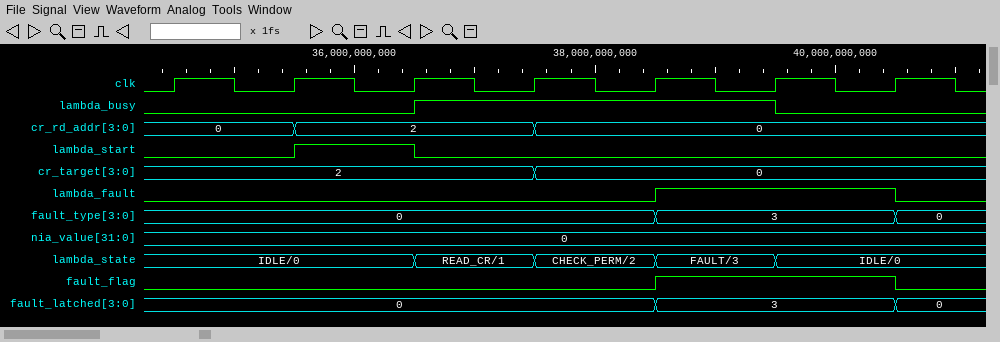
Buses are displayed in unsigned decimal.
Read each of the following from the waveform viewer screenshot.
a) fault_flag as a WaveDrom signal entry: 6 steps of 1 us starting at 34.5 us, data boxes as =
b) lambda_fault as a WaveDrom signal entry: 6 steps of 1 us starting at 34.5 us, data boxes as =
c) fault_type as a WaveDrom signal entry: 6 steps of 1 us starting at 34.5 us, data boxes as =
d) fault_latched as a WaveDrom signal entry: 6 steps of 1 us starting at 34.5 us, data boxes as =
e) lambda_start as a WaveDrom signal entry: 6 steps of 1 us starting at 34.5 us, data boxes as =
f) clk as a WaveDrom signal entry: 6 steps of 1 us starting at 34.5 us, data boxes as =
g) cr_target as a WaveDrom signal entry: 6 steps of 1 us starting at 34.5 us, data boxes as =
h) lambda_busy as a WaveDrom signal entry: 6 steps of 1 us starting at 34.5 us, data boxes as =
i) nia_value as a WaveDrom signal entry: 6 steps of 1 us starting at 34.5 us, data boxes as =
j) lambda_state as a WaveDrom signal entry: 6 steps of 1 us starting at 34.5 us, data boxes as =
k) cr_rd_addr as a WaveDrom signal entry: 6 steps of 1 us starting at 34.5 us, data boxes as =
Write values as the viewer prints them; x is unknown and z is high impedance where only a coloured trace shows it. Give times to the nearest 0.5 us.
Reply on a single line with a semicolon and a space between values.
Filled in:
{name: 'fault_flag', wave: '0...1.'}; {name: 'lambda_fault', wave: '0...1.'}; {name: 'fault_type', wave: '=...=.', data: '0 3'}; {name: 'fault_latched', wave: '=...=.', data: '0 3'}; {name: 'lambda_start', wave: '010...'}; {name: 'clk', wave: 'p.....'}; {name: 'cr_target', wave: '=..=..', data: '2 0'}; {name: 'lambda_busy', wave: '0.1..0'}; {name: 'nia_value', wave: '=.....', data: '0'}; {name: 'lambda_state', wave: '=.====', data: 'IDLE/0 READ_CR/1 CHECK_PERM/2 FAULT/3 IDLE/0'}; {name: 'cr_rd_addr', wave: '==.=..', data: '0 2 0'}
